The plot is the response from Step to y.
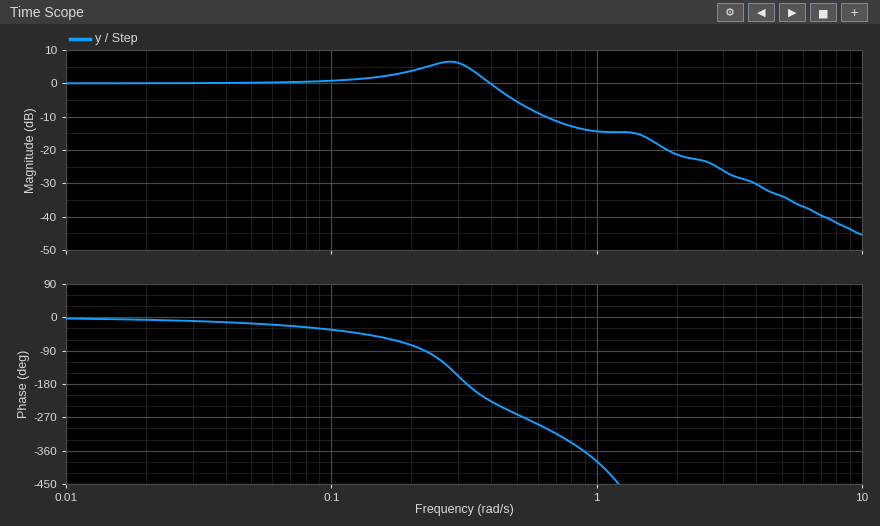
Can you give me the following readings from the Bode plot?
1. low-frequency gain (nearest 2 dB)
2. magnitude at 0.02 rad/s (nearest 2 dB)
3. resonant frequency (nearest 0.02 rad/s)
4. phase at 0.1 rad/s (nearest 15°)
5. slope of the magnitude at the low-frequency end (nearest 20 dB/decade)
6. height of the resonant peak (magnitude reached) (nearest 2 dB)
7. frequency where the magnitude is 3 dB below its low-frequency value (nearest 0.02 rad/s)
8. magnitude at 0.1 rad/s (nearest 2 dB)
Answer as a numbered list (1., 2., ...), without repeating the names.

1. 0 dB
2. 0 dB
3. 0.28 rad/s
4. -30°
5. 0 dB/decade
6. 6 dB
7. 0.44 rad/s
8. 0 dB
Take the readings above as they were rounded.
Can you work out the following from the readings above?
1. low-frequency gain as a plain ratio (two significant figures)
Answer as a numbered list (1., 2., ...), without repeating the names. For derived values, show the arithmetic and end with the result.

1. 10^(0 / 20) = 1.0
